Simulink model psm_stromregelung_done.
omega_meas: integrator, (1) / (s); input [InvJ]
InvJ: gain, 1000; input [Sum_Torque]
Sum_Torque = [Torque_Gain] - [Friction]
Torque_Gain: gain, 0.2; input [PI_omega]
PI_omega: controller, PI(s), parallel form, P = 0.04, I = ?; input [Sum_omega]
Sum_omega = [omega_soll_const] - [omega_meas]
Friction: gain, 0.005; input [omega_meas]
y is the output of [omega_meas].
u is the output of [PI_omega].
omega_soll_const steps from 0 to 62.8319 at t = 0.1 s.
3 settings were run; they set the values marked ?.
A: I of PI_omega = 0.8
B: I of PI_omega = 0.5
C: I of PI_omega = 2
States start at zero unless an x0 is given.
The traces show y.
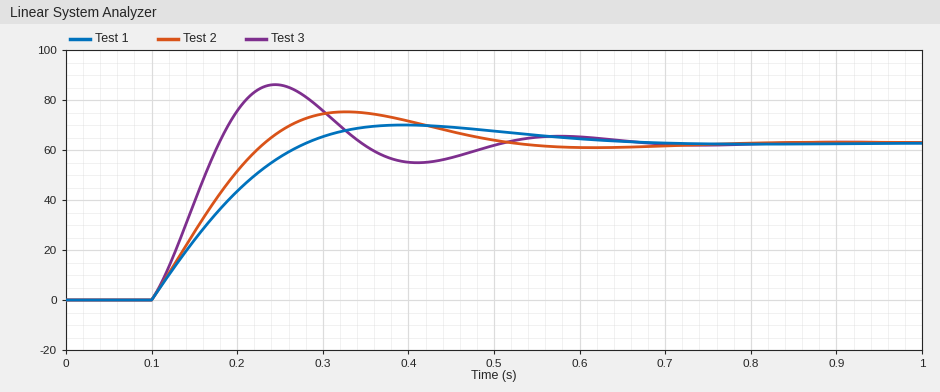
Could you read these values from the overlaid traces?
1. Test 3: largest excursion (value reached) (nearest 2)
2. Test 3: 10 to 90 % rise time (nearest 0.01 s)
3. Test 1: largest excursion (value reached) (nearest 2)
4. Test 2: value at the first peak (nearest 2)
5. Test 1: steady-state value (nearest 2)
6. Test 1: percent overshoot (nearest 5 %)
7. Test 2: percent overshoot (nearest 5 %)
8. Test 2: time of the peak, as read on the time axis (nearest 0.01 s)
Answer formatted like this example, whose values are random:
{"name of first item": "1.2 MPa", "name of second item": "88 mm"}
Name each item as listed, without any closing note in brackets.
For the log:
{"Test 3: largest excursion (value reached)": "86", "Test 3: 10 to 90 % rise time": "0.06 s", "Test 1: largest excursion (value reached)": "70", "Test 2: value at the first peak": "76", "Test 1: steady-state value": "62", "Test 1: percent overshoot": "10 %", "Test 2: percent overshoot": "20 %", "Test 2: time of the peak, as read on the time axis": "0.33 s"}
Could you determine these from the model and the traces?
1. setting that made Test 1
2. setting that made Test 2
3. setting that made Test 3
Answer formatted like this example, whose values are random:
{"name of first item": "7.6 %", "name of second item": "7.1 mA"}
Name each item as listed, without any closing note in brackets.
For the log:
{"setting that made Test 1": "B", "setting that made Test 2": "A", "setting that made Test 3": "C"}
